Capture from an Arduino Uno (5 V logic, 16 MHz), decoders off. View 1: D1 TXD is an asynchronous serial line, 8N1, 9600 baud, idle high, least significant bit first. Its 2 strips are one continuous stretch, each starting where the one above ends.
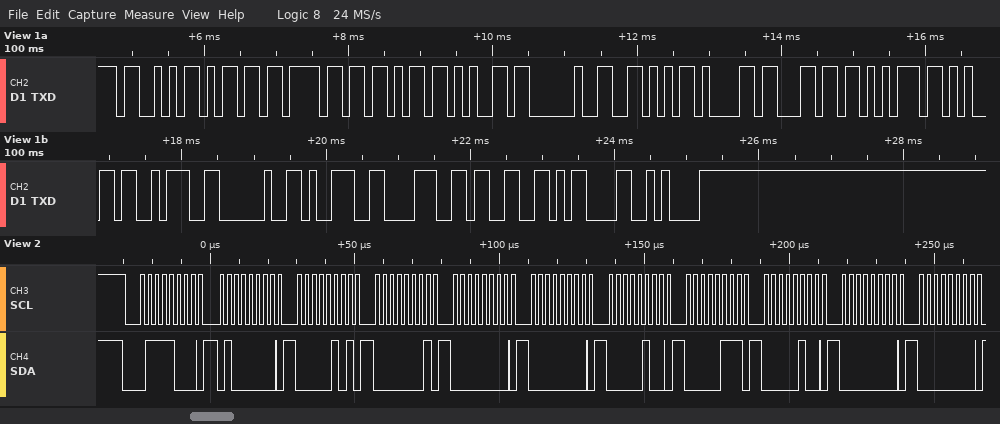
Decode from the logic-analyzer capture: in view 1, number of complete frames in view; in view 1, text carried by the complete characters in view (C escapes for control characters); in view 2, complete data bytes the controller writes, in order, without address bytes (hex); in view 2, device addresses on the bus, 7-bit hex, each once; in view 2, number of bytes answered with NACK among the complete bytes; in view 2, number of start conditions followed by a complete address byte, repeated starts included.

18
"Smoke Value: 983\r\n"
40 05 01 00 00 04 07 04 00 00
0x3C
0
1
